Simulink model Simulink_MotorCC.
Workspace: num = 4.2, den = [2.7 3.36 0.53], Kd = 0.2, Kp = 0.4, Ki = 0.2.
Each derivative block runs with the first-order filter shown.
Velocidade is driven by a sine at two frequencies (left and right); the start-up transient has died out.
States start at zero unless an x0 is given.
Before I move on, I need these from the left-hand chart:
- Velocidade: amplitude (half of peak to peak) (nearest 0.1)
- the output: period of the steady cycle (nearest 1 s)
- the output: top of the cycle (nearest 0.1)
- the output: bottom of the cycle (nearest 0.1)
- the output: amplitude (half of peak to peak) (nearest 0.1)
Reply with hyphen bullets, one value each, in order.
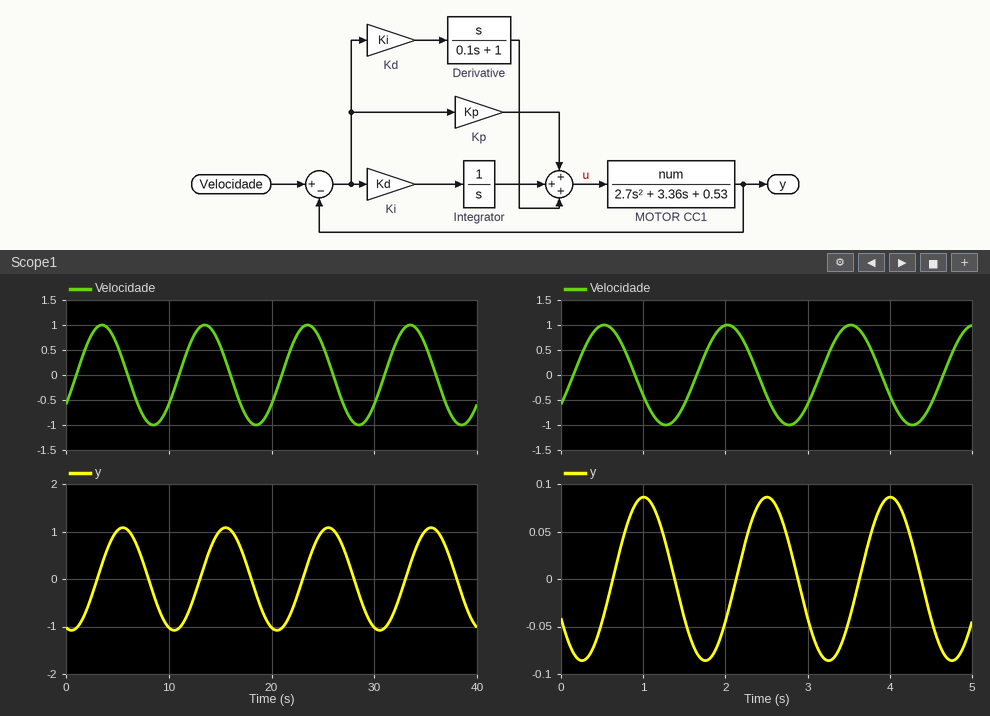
- 1.0
- 10 s
- 1.1
- -1.1
- 1.1
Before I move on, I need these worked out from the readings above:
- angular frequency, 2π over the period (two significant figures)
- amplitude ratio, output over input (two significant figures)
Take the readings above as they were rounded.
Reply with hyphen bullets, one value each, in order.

- 0.63 rad/s
- 1.1
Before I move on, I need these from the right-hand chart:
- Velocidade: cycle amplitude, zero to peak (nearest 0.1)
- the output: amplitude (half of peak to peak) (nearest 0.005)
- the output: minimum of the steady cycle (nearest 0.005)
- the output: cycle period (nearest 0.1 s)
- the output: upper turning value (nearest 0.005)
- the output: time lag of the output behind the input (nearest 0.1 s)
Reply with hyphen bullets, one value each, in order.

- 1.0
- 0.085
- -0.085
- 1.5 s
- 0.085
- 0.5 s
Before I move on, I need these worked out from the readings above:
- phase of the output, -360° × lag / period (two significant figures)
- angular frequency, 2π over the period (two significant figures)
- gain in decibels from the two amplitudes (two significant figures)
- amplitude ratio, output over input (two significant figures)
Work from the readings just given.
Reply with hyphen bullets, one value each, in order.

- -120°
- 4.2 rad/s
- -21 dB
- 0.085
